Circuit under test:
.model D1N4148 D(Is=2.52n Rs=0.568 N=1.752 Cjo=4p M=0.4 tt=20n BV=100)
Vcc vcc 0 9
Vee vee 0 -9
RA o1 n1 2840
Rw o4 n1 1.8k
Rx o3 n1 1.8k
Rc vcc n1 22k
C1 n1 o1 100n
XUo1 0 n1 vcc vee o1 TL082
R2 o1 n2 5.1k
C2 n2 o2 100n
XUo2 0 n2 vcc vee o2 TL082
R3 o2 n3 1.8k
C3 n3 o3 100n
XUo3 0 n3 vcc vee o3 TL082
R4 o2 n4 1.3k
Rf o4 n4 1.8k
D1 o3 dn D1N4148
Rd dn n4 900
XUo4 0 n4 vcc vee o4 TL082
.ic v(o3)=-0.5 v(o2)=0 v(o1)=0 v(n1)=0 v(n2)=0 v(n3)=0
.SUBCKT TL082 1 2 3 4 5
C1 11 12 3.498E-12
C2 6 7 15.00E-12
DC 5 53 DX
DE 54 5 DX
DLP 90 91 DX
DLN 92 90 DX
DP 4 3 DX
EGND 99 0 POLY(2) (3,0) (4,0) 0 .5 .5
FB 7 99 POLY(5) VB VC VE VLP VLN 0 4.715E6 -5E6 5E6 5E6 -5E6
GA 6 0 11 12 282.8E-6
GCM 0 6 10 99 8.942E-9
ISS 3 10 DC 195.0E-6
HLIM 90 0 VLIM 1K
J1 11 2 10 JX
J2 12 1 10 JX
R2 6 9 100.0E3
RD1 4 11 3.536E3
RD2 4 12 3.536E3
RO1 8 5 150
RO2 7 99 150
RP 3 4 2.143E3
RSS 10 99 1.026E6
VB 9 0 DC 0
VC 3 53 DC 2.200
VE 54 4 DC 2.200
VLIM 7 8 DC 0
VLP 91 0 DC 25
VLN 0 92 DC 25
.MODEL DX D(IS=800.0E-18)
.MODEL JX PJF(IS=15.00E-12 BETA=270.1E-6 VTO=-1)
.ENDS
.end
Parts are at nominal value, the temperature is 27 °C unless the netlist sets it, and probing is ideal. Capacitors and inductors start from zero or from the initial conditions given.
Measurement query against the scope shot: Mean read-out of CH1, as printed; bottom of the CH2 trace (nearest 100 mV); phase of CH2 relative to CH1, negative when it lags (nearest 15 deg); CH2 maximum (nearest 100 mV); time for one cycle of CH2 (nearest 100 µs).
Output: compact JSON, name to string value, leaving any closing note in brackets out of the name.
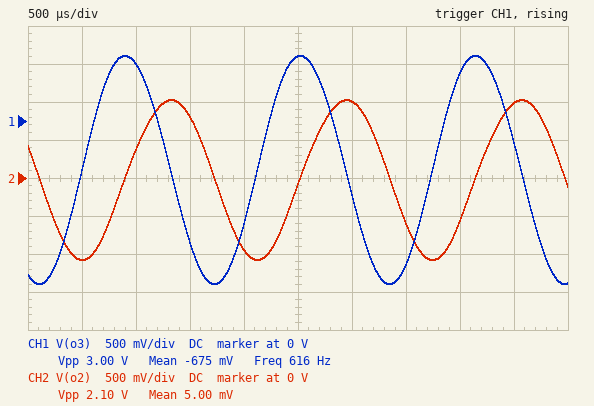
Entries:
{"Mean read-out of CH1, as printed": "-675 mV", "bottom of the CH2 trace": "-1.1 V", "phase of CH2 relative to CH1, negative when it lags": "-90 deg", "CH2 maximum": "1.0 V", "time for one cycle of CH2": "1.6 ms"}
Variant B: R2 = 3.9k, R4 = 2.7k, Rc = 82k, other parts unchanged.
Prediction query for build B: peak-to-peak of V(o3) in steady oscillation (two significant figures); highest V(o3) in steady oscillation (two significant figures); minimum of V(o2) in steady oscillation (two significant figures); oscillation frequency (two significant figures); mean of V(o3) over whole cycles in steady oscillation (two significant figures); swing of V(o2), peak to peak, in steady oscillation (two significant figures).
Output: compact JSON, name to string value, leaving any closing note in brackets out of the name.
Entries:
{"peak-to-peak of V(o3) in steady oscillation": "800 mV", "highest V(o3) in steady oscillation": "7.5 V", "minimum of V(o2) in steady oscillation": "-800 mV", "oscillation frequency": "350 Hz", "mean of V(o3) over whole cycles in steady oscillation": "7.3 V", "swing of V(o2), peak to peak, in steady oscillation": "1.1 V"}
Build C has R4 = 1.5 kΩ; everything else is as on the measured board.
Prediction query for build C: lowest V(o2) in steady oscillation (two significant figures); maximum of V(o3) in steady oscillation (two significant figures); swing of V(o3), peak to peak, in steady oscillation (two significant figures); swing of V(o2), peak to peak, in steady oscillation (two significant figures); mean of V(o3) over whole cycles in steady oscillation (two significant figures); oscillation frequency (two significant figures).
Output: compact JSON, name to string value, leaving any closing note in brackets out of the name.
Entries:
{"lowest V(o2) in steady oscillation": "-1.2 V", "maximum of V(o3) in steady oscillation": "1.2 V", "swing of V(o3), peak to peak, in steady oscillation": "3.4 V", "swing of V(o2), peak to peak, in steady oscillation": "2.2 V", "mean of V(o3) over whole cycles in steady oscillation": "-500 mV", "oscillation frequency": "570 Hz"}
